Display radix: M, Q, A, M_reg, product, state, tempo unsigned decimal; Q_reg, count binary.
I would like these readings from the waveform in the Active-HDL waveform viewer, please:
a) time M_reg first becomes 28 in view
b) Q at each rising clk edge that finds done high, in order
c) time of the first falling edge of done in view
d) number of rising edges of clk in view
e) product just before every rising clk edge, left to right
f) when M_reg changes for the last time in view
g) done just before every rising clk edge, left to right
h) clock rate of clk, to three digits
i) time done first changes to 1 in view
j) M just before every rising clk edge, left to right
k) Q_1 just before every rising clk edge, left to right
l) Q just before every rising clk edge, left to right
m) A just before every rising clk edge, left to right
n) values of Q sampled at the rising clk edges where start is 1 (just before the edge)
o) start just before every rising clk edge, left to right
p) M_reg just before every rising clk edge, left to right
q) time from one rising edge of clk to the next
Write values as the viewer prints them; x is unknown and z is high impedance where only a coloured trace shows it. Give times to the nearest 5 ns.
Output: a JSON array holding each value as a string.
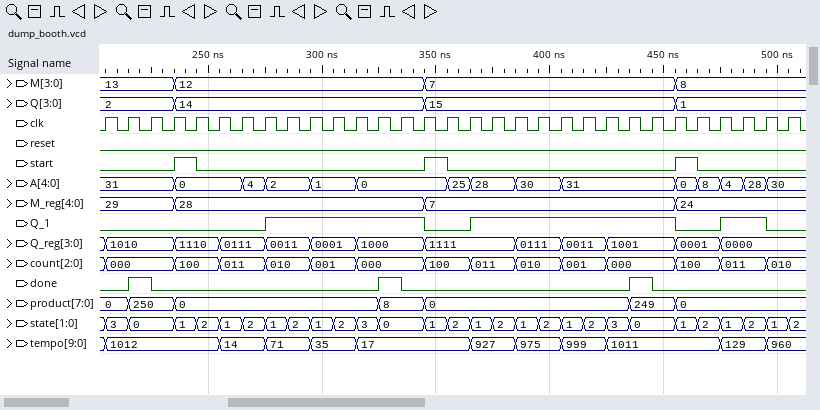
["235 ns", "2, 14, 15", "225 ns", "31", "0, 0, 250, 250, 0, 0, 0, 0, 0, 0, 0, 0, 0, 8, 8, 0, 0, 0, 0, 0, 0, 0, 0, 0, 249, 249, 0, 0, 0, 0, 0", "455 ns", "0 0 1 0 0 0 0 0 0 0 0 0 0 1 0 0 0 0 0 0 0 0 0 0 1 0 0 0 0 0 0", "100 MHz", "215 ns", "13, 13, 13, 13, 12, 12, 12, 12, 12, 12, 12, 12, 12, 12, 12, 7, 7, 7, 7, 7, 7, 7, 7, 7, 7, 7, 8, 8, 8, 8, 8", "0 0 0 0 0 0 0 0 1 1 1 1 1 1 1 0 0 1 1 1 1 1 1 1 1 1 0 0 1 1 0", "2, 2, 2, 2, 14, 14, 14, 14, 14, 14, 14, 14, 14, 14, 14, 15, 15, 15, 15, 15, 15, 15, 15, 15, 15, 15, 1, 1, 1, 1, 1", "31, 31, 31, 31, 0, 0, 0, 4, 2, 2, 1, 1, 0, 0, 0, 0, 25, 28, 28, 30, 30, 31, 31, 31, 31, 31, 0, 8, 4, 28, 30", "14, 15, 1", "0 0 0 0 1 0 0 0 0 0 0 0 0 0 0 1 0 0 0 0 0 0 0 0 0 0 1 0 0 0 0", "29, 29, 29, 29, 28, 28, 28, 28, 28, 28, 28, 28, 28, 28, 28, 7, 7, 7, 7, 7, 7, 7, 7, 7, 7, 7, 24, 24, 24, 24, 24", "10 ns"]
